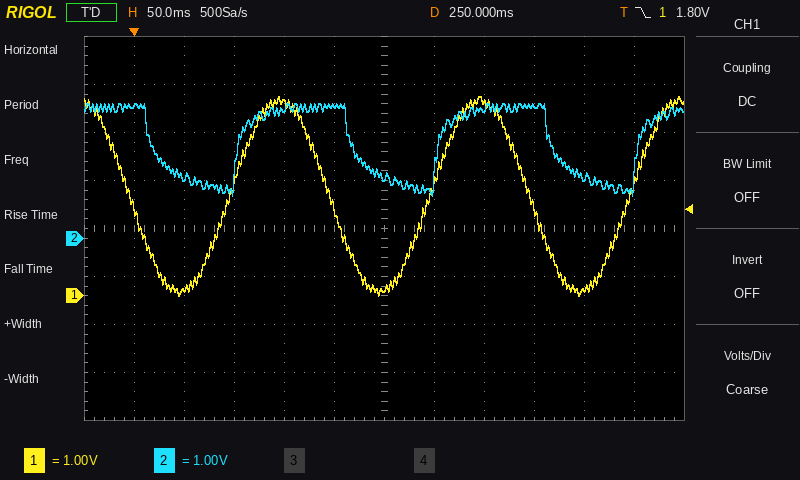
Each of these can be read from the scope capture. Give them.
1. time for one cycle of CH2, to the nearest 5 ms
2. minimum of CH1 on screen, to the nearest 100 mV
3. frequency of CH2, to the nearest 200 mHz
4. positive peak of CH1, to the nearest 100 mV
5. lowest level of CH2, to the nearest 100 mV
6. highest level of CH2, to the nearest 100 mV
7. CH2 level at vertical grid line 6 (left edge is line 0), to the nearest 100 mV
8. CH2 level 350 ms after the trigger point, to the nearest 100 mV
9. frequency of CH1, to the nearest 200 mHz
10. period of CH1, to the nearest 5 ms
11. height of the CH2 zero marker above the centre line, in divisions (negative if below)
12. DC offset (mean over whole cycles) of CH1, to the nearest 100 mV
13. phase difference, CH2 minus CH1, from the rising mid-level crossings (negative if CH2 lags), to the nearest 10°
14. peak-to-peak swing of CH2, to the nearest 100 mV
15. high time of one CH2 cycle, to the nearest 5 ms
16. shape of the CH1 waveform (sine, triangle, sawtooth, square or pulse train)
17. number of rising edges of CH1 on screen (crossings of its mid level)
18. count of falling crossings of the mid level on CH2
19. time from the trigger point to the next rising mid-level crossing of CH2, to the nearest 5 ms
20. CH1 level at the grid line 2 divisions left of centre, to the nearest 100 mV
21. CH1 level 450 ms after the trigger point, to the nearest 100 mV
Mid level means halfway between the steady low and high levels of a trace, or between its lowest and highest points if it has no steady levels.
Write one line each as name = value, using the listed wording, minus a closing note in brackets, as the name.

time for one cycle of CH2, to the nearest 5 ms = 200 ms
minimum of CH1 on screen, to the nearest 100 mV = 0.0 V
frequency of CH2, to the nearest 200 mHz = 5.0 Hz
positive peak of CH1, to the nearest 100 mV = 4.2 V
lowest level of CH2, to the nearest 100 mV = 900 mV
highest level of CH2, to the nearest 100 mV = 2.8 V
CH2 level at vertical grid line 6 (left edge is line 0), to the nearest 100 mV = 1.3 V
CH2 level 350 ms after the trigger point, to the nearest 100 mV = 2.7 V
frequency of CH1, to the nearest 200 mHz = 5.0 Hz
period of CH1, to the nearest 5 ms = 200 ms
height of the CH2 zero marker above the centre line, in divisions = -0.2 div
DC offset (mean over whole cycles) of CH1, to the nearest 100 mV = 2.1 V
phase difference, CH2 minus CH1, from the rising mid-level crossings (negative if CH2 lags), to the nearest 10° = -10°
peak-to-peak swing of CH2, to the nearest 100 mV = 1.9 V
high time of one CH2 cycle, to the nearest 5 ms = 115 ms
shape of the CH1 waveform = sine
number of rising edges of CH1 on screen = 3
count of falling crossings of the mid level on CH2 = 3
time from the trigger point to the next rising mid-level crossing of CH2, to the nearest 5 ms = 105 ms
CH1 level at the grid line 2 divisions left of centre, to the nearest 100 mV = 4.0 V
CH1 level 450 ms after the trigger point, to the nearest 100 mV = 200 mV
